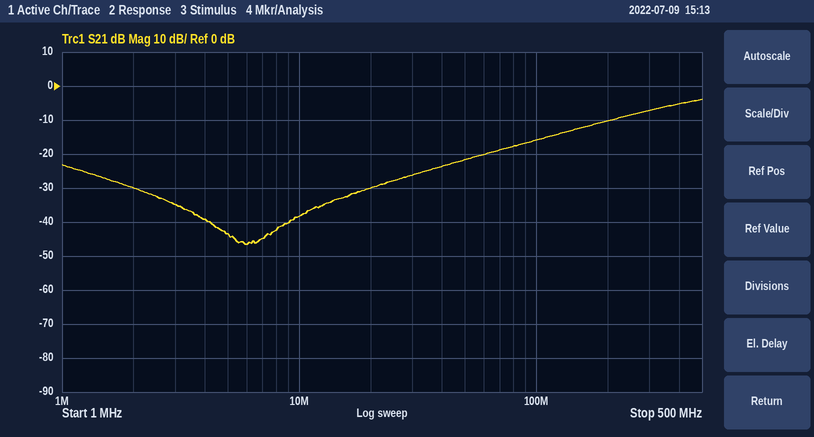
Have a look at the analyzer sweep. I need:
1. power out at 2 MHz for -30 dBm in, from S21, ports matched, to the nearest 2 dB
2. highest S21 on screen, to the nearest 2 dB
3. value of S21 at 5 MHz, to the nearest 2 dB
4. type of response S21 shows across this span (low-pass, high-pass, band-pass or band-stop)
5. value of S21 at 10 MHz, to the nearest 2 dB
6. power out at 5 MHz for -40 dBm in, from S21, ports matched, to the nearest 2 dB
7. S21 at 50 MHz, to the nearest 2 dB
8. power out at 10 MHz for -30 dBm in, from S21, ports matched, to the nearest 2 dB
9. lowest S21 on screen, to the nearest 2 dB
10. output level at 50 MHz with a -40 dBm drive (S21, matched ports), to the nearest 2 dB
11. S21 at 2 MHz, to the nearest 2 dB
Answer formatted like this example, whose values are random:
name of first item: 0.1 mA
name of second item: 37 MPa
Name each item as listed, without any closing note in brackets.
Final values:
power out at 2 MHz for -30 dBm in, from S21, ports matched, to the nearest 2 dB: -60 dBm
highest S21 on screen, to the nearest 2 dB: -4 dB
value of S21 at 5 MHz, to the nearest 2 dB: -44 dB
type of response S21 shows across this span: high-pass
value of S21 at 10 MHz, to the nearest 2 dB: -38 dB
power out at 5 MHz for -40 dBm in, from S21, ports matched, to the nearest 2 dB: -84 dBm
S21 at 50 MHz, to the nearest 2 dB: -22 dB
power out at 10 MHz for -30 dBm in, from S21, ports matched, to the nearest 2 dB: -68 dBm
lowest S21 on screen, to the nearest 2 dB: -46 dB
output level at 50 MHz with a -40 dBm drive (S21, matched ports), to the nearest 2 dB: -62 dBm
S21 at 2 MHz, to the nearest 2 dB: -30 dB
